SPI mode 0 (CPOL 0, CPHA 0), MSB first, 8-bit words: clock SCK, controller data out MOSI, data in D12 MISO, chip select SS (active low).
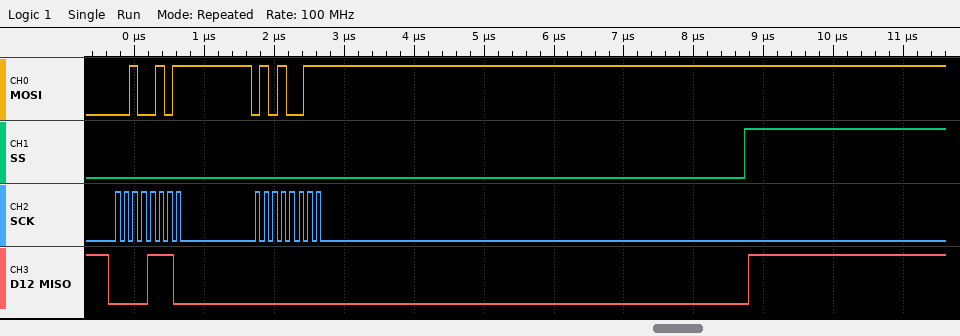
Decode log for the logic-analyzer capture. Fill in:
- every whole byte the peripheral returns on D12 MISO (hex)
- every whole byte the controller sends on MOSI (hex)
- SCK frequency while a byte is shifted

0E 00
25 53
8 MHz
